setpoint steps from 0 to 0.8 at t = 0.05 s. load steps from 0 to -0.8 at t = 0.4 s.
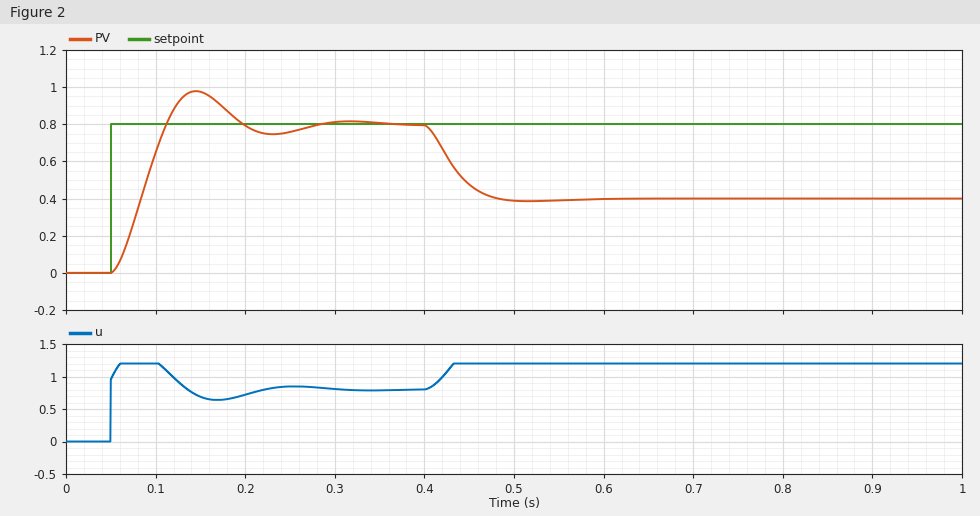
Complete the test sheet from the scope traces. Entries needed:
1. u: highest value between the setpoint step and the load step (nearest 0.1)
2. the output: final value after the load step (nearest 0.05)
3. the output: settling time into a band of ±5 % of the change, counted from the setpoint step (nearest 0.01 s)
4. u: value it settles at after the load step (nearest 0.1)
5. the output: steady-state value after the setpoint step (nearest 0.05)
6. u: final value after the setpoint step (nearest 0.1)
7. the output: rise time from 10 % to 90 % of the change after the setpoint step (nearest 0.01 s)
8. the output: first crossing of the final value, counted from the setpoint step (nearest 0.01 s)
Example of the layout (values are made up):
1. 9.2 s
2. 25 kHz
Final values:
1. 1.2
2. 0.40
3. 0.20 s
4. 1.2
5. 0.80
6. 0.8
7. 0.04 s
8. 0.06 s
